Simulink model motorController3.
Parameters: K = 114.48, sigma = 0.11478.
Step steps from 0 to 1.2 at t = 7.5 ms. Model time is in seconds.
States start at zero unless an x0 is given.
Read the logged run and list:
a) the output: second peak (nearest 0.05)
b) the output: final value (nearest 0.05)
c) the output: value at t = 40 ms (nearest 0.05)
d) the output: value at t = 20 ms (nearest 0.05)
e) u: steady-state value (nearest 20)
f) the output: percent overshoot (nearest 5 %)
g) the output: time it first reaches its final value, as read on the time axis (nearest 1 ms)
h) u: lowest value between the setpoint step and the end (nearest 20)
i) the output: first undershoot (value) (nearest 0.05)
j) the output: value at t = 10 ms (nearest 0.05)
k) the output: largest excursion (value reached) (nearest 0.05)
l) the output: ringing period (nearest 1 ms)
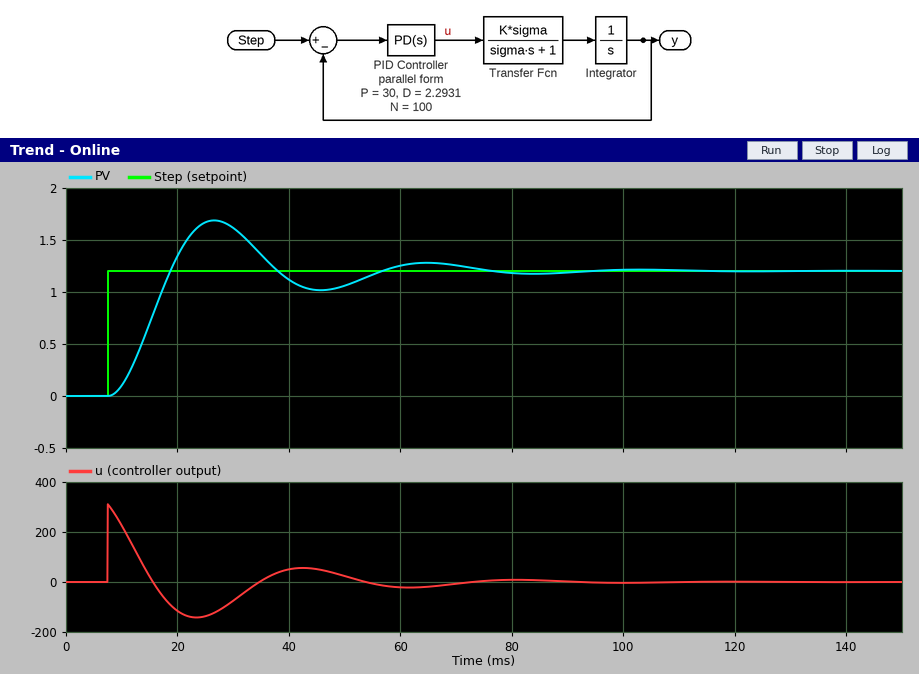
1.30
1.20
1.10
1.35
0
40 %
19 ms
-140
1.00
0.10
1.70
38 ms
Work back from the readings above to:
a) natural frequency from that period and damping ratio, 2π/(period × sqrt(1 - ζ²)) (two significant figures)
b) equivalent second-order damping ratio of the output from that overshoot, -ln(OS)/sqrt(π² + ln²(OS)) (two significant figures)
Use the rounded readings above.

0.17 rad/ms
0.28
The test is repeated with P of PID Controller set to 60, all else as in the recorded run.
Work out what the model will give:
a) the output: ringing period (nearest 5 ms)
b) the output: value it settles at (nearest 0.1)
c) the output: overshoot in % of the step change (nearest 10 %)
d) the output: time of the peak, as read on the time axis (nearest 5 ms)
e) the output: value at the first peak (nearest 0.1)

35 ms
1.2
50 %
25 ms
1.8
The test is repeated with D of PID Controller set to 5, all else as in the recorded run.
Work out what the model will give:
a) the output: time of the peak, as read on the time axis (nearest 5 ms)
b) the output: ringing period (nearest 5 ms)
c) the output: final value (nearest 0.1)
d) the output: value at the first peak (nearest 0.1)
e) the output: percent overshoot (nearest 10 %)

20 ms
25 ms
1.2
1.8
50 %
